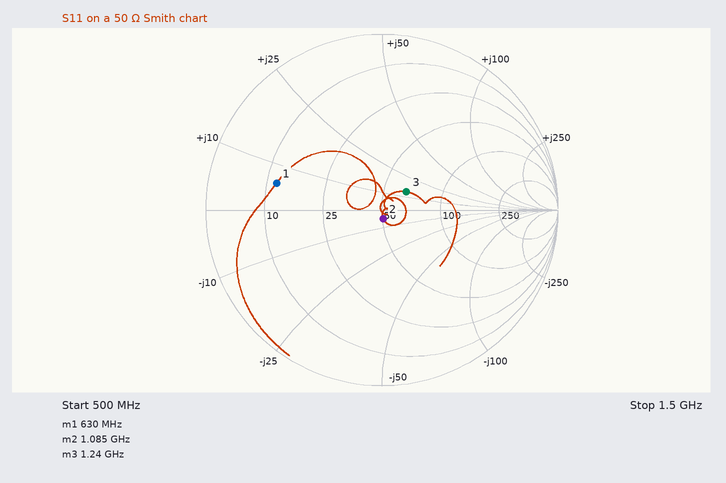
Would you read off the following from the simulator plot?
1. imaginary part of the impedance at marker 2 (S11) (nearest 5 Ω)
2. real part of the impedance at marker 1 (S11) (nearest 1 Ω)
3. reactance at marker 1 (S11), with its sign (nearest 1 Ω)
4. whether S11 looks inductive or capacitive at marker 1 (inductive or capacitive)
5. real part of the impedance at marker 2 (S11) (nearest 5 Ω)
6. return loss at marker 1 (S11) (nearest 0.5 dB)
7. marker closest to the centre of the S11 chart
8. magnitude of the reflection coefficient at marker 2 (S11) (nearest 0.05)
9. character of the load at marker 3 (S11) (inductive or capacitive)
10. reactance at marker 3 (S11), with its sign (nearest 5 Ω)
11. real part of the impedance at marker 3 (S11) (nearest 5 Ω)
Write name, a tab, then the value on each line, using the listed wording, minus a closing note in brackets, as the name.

imaginary part of the impedance at marker 2 (S11)	-5 Ω
real part of the impedance at marker 1 (S11)	12 Ω
reactance at marker 1 (S11), with its sign	+6 Ω
whether S11 looks inductive or capacitive at marker 1	inductive
real part of the impedance at marker 2 (S11)	50 Ω
return loss at marker 1 (S11)	4.0 dB
marker closest to the centre of the S11 chart	marker 2
magnitude of the reflection coefficient at marker 2 (S11)	0.05
character of the load at marker 3 (S11)	inductive
reactance at marker 3 (S11), with its sign	+15 Ω
real part of the impedance at marker 3 (S11)	65 Ω
